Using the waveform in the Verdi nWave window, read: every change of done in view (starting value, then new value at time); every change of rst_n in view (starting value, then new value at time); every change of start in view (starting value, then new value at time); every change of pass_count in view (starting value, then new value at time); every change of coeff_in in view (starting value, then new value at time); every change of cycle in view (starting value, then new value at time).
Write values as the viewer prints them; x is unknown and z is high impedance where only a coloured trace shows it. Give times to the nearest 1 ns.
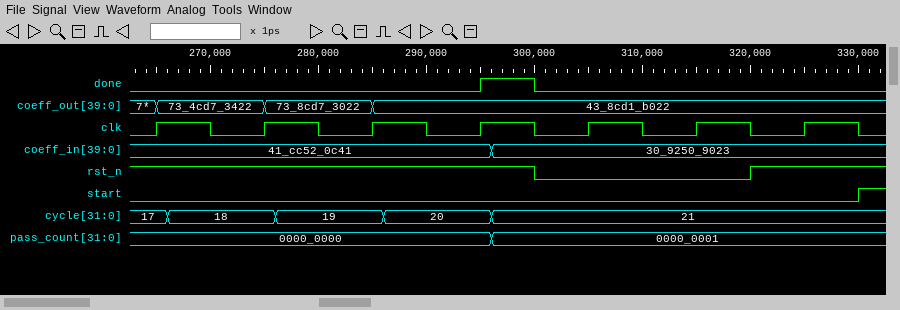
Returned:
0, 1 at 295 ns, 0 at 300 ns
1, 0 at 300 ns, 1 at 320 ns
0, 1 at 330 ns
0000_0000, 0000_0001 at 296 ns
41_cc52_0c41, 30_9250_9023 at 296 ns
17, 18 at 266 ns, 19 at 276 ns, 20 at 286 ns, 21 at 296 ns
